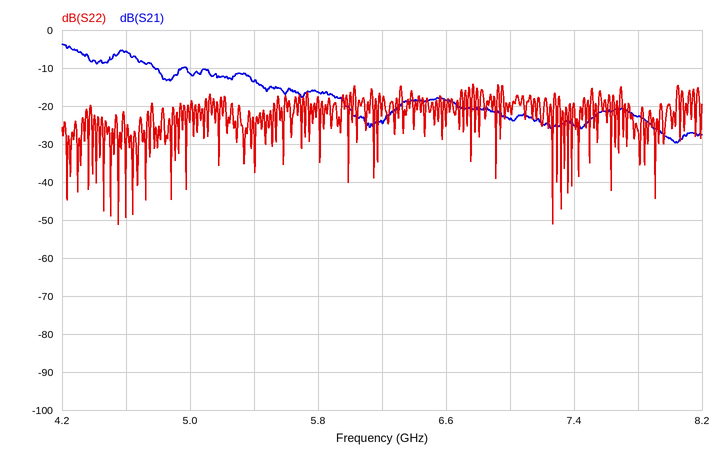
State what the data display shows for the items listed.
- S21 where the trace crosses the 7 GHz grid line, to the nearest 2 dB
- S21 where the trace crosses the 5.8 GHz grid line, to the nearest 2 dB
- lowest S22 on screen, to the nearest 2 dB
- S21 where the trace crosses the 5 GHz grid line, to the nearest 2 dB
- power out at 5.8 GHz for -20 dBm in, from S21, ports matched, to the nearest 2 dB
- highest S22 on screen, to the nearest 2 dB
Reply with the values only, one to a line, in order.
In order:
-24 dB
-16 dB
-52 dB
-12 dB
-36 dBm
-14 dB
